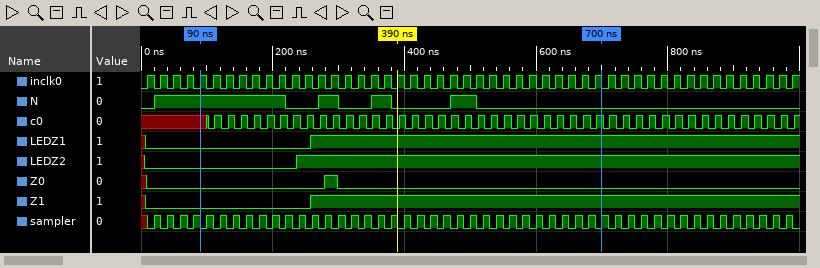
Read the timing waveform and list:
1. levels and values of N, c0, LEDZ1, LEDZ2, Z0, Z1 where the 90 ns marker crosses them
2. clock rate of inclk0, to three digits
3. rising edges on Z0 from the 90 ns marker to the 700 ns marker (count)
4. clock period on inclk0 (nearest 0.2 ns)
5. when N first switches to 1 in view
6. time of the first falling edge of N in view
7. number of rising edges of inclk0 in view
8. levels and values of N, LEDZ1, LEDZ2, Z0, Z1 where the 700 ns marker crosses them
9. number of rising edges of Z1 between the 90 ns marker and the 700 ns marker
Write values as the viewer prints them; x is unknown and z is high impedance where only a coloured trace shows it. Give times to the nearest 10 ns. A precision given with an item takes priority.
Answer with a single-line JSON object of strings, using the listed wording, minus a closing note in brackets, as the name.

{"levels and values of N, c0, LEDZ1, LEDZ2, Z0, Z1 where the 90 ns marker crosses them": "N=1, c0=x, LEDZ1=0, LEDZ2=0, Z0=0, Z1=0", "clock rate of inclk0, to three digits": "50.0 MHz", "rising edges on Z0 from the 90 ns marker to the 700 ns marker": "1", "clock period on inclk0": "20 ns", "when N first switches to 1 in view": "20 ns", "time of the first falling edge of N in view": "220 ns", "number of rising edges of inclk0 in view": "50", "levels and values of N, LEDZ1, LEDZ2, Z0, Z1 where the 700 ns marker crosses them": "N=0, LEDZ1=1, LEDZ2=1, Z0=0, Z1=1", "number of rising edges of Z1 between the 90 ns marker and the 700 ns marker": "1"}
